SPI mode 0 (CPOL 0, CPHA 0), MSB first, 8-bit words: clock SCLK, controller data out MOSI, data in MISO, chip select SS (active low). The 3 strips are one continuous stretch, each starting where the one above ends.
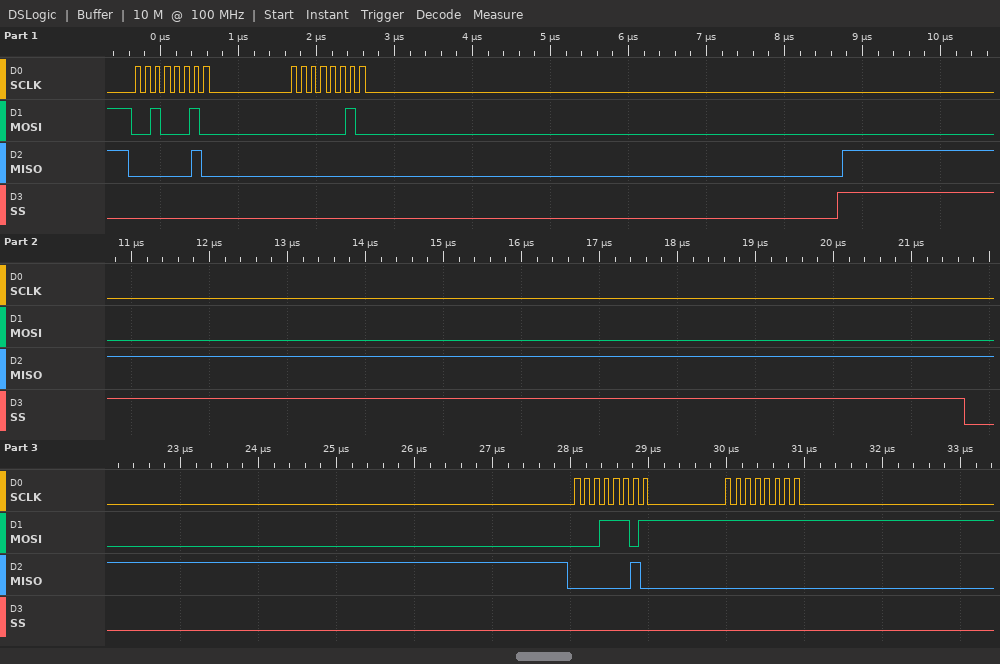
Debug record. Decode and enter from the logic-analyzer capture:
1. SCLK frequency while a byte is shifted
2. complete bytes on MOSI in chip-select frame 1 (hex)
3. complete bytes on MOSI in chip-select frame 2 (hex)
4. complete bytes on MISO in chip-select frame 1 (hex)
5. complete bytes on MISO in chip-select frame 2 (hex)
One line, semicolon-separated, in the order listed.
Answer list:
8 MHz; 22 02; 1D FF; 02 00; 02 00
